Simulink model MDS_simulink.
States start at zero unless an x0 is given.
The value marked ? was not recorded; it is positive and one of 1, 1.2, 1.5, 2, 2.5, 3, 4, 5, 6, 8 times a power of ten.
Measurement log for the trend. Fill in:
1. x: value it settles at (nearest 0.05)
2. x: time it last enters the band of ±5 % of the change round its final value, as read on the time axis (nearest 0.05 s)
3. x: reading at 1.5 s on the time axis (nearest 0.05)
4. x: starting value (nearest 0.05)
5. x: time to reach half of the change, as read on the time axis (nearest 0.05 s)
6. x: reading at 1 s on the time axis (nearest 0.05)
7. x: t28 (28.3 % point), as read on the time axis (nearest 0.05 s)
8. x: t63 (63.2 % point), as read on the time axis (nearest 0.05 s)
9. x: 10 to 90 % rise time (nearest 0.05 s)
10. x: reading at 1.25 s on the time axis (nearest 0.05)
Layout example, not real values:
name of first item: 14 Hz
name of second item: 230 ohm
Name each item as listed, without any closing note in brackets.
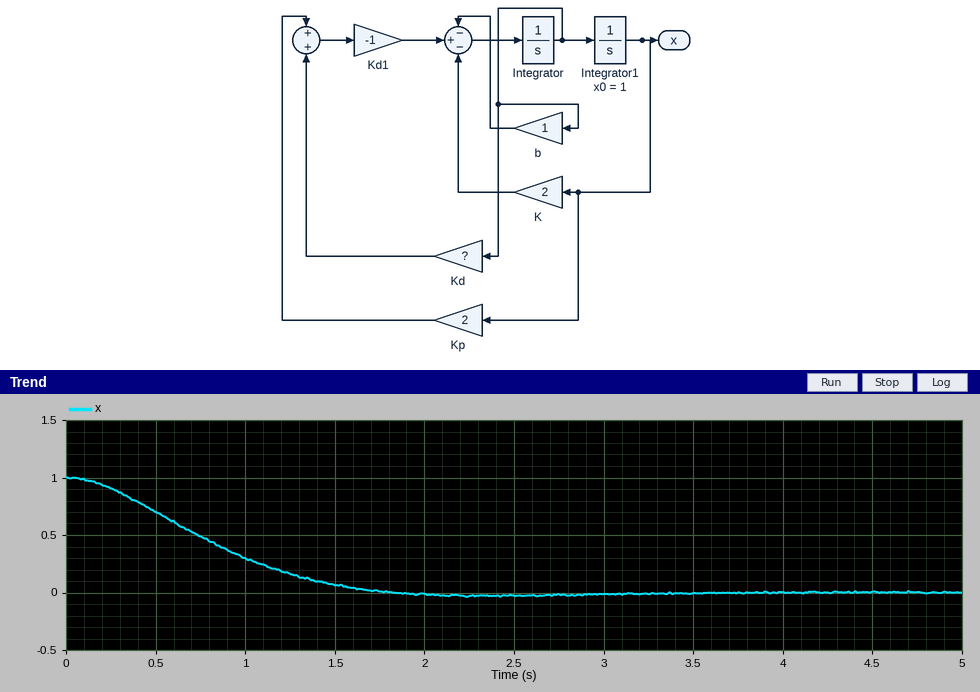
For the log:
x: value it settles at: 0.00
x: time it last enters the band of ±5 % of the change round its final value, as read on the time axis: 1.55 s
x: reading at 1.5 s on the time axis: 0.05
x: starting value: 1.00
x: time to reach half of the change, as read on the time axis: 0.75 s
x: reading at 1 s on the time axis: 0.30
x: t28 (28.3 % point), as read on the time axis: 0.50 s
x: t63 (63.2 % point), as read on the time axis: 0.90 s
x: 10 to 90 % rise time: 1.15 s
x: reading at 1.25 s on the time axis: 0.15
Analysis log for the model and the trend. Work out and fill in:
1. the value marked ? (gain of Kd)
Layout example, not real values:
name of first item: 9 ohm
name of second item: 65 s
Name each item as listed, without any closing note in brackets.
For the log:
the value marked ?: 2
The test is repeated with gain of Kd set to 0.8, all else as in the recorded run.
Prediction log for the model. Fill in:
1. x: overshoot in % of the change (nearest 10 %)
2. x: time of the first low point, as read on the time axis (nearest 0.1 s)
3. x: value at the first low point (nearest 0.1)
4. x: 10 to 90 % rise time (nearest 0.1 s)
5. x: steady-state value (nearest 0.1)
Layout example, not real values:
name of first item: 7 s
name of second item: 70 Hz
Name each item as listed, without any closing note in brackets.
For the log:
x: overshoot in % of the change: 20 %
x: time of the first low point, as read on the time axis: 1.8 s
x: value at the first low point: -0.2
x: 10 to 90 % rise time: 0.8 s
x: steady-state value: 0.0
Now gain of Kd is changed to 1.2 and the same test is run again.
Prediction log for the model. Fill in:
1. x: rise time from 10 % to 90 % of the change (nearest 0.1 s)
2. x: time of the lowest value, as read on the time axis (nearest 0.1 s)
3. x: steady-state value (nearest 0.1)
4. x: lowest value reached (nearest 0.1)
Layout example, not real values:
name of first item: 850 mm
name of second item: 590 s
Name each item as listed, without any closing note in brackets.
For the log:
x: rise time from 10 % to 90 % of the change: 0.9 s
x: time of the lowest value, as read on the time axis: 1.9 s
x: steady-state value: 0.0
x: lowest value reached: -0.1
